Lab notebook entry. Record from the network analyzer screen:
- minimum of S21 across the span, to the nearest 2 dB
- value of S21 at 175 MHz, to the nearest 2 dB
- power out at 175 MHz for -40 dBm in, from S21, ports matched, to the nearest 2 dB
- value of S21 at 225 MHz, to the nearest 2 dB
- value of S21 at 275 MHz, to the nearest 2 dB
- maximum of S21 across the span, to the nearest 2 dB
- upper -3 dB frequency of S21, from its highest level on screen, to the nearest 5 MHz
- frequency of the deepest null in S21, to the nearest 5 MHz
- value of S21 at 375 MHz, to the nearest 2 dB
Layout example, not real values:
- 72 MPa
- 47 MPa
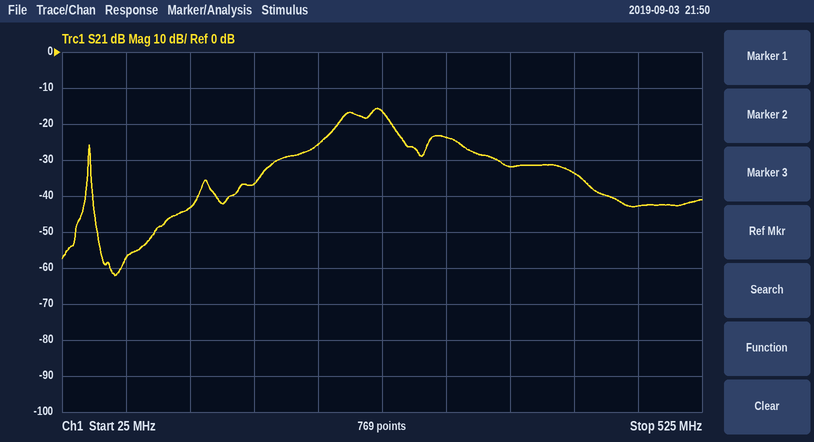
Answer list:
- -62 dB
- -36 dB
- -76 dBm
- -26 dB
- -16 dB
- -16 dB
- 280 MHz
- 65 MHz
- -32 dB
